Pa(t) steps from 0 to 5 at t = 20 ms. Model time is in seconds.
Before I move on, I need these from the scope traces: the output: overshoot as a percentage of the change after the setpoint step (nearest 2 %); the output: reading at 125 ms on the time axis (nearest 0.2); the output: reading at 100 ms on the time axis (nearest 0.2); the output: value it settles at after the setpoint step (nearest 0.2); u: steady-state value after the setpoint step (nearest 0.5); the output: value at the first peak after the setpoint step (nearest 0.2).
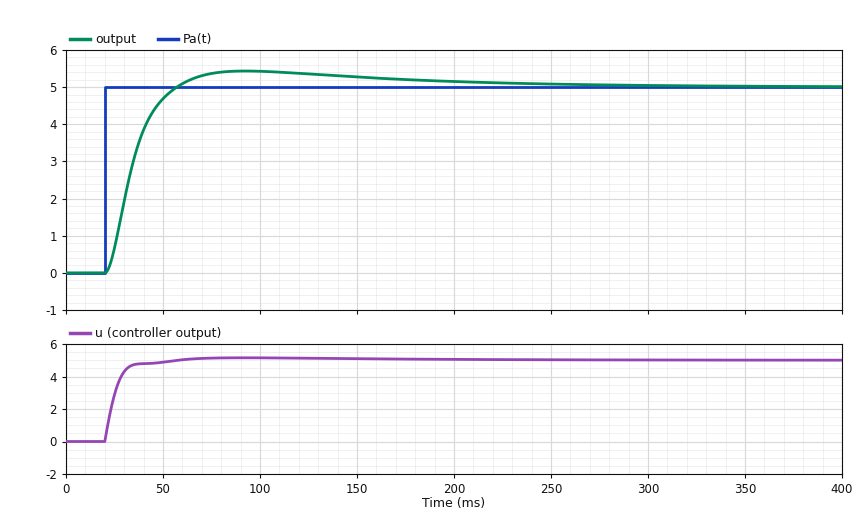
8 %
5.4
5.4
5.0
5.0
5.4
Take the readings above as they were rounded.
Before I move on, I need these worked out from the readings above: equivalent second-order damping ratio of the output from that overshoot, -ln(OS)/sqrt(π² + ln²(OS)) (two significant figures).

0.63
